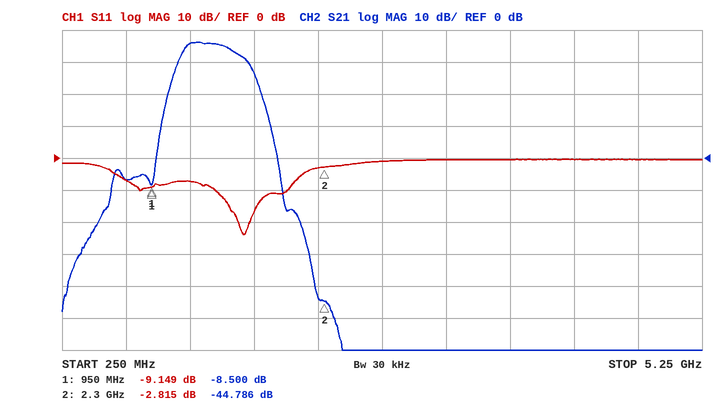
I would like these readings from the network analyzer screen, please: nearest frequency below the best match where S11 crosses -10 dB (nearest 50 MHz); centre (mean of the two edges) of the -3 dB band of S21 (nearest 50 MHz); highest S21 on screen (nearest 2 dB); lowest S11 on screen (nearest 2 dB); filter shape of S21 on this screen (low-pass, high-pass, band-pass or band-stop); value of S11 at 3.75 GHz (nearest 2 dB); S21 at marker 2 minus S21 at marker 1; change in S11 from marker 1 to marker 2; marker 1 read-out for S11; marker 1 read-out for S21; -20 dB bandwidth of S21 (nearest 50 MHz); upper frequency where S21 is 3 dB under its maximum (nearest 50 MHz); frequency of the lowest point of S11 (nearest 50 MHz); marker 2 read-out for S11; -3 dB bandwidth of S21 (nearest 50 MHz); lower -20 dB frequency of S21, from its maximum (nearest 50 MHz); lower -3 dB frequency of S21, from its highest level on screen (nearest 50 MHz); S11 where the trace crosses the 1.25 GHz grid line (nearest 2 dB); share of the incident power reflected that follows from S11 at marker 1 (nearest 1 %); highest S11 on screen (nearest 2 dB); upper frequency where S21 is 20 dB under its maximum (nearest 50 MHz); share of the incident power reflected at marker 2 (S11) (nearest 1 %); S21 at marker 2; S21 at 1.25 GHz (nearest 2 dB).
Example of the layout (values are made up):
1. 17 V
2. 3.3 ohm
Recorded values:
1. 1.45 GHz
2. 1.40 GHz
3. 36 dB
4. -24 dB
5. band-pass
6. 0 dB
7. -36.286 dB
8. 6.334 dB
9. -9.149 dB
10. -8.500 dB
11. 800 MHz
12. 1.60 GHz
13. 1.65 GHz
14. -2.815 dB
15. 400 MHz
16. 1.05 GHz
17. 1.20 GHz
18. -8 dB
19. 12 %
20. 0 dB
21. 1.85 GHz
22. 52 %
23. -44.786 dB
24. 36 dB
